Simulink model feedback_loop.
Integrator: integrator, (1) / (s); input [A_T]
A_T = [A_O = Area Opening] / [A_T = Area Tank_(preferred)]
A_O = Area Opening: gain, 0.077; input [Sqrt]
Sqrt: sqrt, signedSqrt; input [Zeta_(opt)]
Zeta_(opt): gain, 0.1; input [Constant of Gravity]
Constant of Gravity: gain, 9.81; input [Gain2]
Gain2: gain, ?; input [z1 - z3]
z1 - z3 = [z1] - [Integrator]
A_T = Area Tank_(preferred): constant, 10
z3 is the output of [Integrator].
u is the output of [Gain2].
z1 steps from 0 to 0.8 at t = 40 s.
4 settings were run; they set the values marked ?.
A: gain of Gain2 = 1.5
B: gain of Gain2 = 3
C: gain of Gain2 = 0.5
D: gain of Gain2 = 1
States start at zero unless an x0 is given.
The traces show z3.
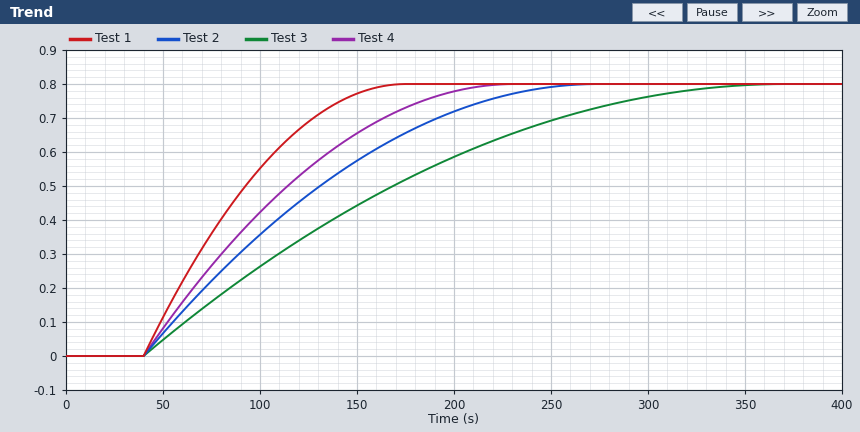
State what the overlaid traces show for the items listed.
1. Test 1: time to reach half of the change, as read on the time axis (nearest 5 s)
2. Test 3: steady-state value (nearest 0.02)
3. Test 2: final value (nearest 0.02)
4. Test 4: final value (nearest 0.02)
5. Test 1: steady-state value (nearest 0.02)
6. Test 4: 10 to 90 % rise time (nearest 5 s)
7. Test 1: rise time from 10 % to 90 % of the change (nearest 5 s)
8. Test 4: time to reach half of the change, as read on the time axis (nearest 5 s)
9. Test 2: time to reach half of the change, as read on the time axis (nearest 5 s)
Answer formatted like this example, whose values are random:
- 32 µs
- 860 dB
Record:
- 80 s
- 0.80
- 0.80
- 0.80
- 0.80
- 120 s
- 85 s
- 95 s
- 110 s
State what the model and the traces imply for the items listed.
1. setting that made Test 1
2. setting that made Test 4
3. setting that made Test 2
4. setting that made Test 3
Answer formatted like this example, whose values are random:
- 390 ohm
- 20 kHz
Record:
- B
- A
- D
- C
